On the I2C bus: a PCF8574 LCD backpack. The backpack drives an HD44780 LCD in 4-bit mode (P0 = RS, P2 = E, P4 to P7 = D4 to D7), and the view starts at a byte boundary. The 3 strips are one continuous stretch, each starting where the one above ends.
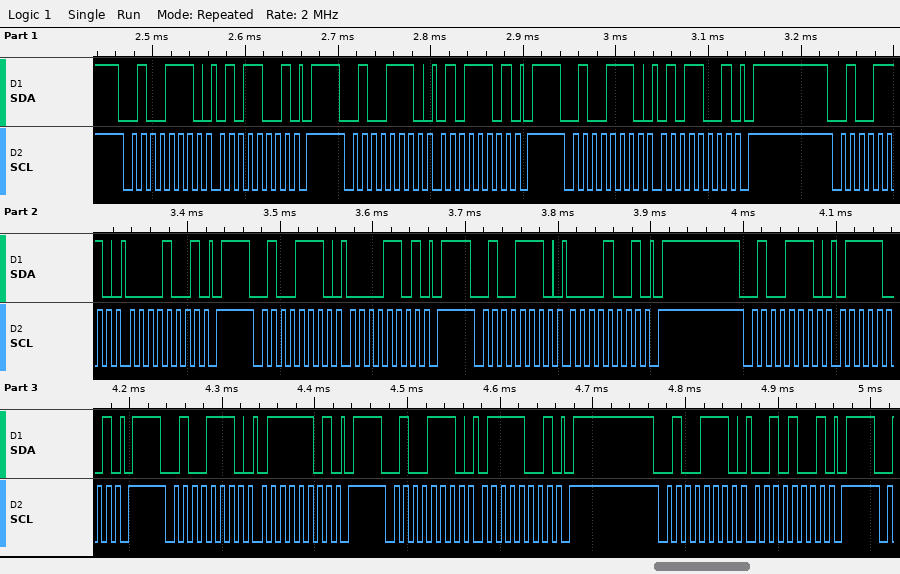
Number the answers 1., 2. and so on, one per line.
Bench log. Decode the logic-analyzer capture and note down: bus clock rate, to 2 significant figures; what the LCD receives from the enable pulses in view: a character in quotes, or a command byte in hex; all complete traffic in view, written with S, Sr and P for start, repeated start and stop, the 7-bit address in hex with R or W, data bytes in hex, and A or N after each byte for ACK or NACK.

1. 100 kHz
2. 'P'
3. S 27W A 59 A P S 27W A 5D A P S 27W A 59 A P S 27W A 09 A P S 27W A 0D A P S 27W A 09 A P S 27W A 79 A P S 27W A 7D A P S 27W A 79 A P S 27W A 29 A P
